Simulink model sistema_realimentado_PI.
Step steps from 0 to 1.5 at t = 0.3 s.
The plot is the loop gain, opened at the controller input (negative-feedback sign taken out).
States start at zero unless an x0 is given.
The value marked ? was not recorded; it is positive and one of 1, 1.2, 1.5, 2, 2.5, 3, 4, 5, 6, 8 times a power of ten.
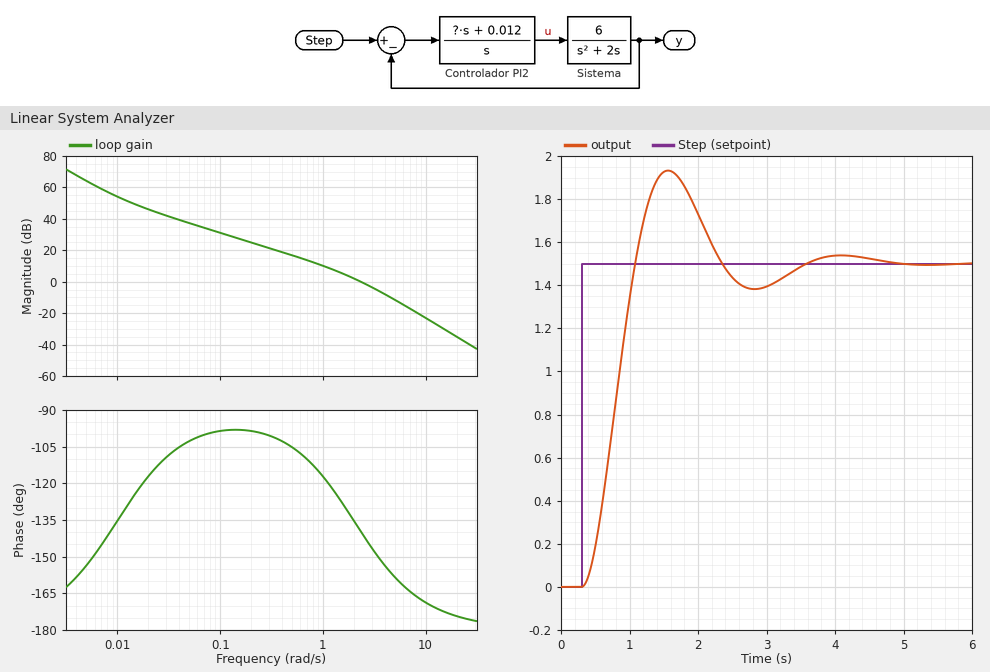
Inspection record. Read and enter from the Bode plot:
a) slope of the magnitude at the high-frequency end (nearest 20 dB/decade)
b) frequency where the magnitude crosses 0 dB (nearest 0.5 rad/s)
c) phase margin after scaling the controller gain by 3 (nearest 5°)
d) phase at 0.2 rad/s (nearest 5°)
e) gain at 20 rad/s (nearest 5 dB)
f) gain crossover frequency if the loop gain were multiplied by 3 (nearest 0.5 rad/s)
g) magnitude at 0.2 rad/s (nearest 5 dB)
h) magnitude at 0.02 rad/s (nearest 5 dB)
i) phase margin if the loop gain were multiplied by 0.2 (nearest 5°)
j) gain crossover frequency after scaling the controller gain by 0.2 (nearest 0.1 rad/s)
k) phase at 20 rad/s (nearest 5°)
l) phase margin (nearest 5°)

-40 dB/decade
2.5 rad/s
25°
-100°
-35 dB
4.5 rad/s
25 dB
45 dB
70°
0.7 rad/s
-175°
40°
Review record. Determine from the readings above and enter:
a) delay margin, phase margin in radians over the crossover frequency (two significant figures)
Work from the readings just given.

0.28 s
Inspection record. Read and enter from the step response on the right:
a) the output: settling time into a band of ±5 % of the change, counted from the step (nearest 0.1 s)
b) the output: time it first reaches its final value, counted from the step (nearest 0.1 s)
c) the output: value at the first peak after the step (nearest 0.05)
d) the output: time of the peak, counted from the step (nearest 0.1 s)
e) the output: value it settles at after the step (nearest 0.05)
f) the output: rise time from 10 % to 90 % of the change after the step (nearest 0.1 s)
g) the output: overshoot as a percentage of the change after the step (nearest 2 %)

2.9 s
0.8 s
1.95
1.3 s
1.50
0.5 s
28 %
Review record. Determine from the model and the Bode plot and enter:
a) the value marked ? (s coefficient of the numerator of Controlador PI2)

1.2
